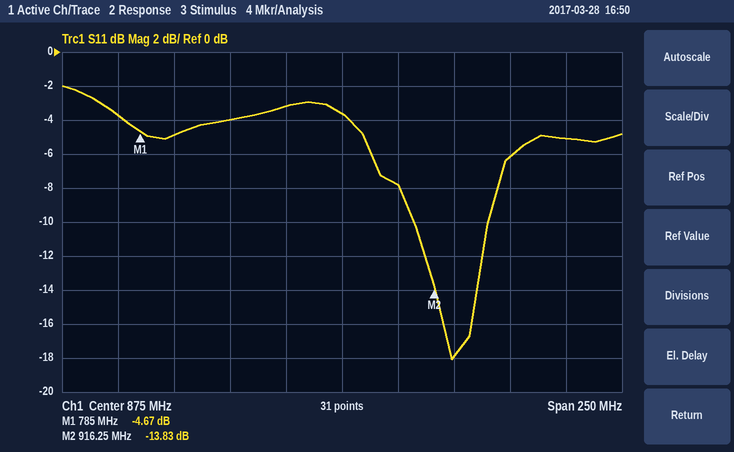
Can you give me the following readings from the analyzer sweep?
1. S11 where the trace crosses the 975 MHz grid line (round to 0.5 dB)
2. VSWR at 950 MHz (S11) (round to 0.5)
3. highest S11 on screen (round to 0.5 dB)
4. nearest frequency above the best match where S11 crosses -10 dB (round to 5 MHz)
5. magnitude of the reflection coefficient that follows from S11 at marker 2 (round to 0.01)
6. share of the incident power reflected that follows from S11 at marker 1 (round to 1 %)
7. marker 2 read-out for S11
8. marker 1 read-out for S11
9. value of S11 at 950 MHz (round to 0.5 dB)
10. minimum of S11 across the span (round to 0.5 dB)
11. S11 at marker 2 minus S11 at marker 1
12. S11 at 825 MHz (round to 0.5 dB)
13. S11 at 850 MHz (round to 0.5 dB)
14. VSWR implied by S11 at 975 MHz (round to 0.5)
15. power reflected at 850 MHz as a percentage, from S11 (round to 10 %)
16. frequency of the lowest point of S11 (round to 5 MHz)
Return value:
-5.0 dB
3.0
-2.0 dB
940 MHz
0.20
34 %
-13.83 dB
-4.67 dB
-6.0 dB
-18.0 dB
-9.16 dB
-4.0 dB
-3.0 dB
3.5
50 %
925 MHz
